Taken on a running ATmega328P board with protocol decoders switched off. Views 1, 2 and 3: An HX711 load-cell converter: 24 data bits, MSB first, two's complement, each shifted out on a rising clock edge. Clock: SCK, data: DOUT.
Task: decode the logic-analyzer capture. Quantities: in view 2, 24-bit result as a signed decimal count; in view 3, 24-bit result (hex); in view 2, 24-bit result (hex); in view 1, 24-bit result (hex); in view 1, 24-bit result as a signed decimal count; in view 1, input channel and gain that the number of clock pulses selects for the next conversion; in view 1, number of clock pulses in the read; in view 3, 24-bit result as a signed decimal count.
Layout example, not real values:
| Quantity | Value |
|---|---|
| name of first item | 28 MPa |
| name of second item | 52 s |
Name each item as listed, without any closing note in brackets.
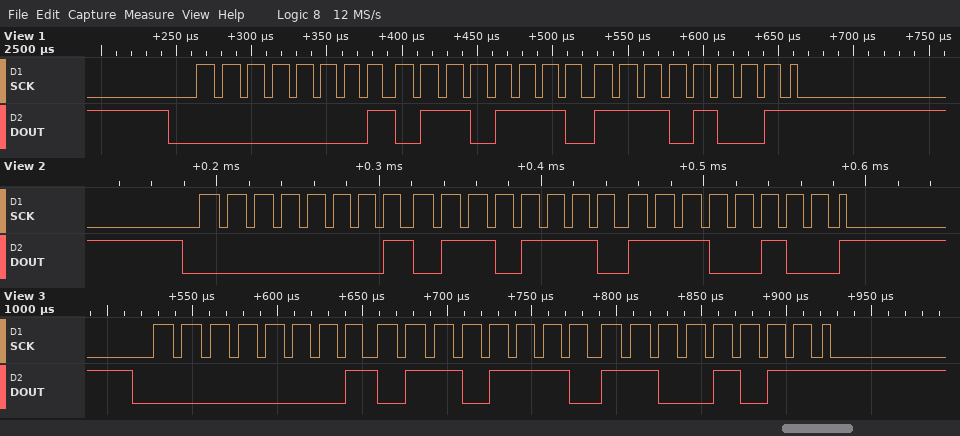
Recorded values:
| Quantity | Value |
|---|---|
| in view 2, 24-bit result as a signed decimal count | 93924 |
| in view 3, 24-bit result | 0x016ECB |
| in view 2, 24-bit result | 0x016EE4 |
| in view 1, 24-bit result | 0x016EE9 |
| in view 1, 24-bit result as a signed decimal count | 93929 |
| in view 1, input channel and gain that the number of clock pulses selects for the next conversion | channel A, gain 128 |
| in view 1, number of clock pulses in the read | 25 |
| in view 3, 24-bit result as a signed decimal count | 93899 |
